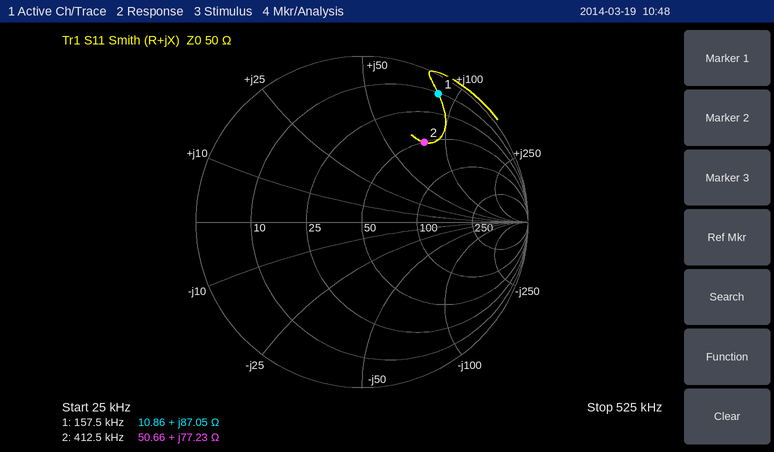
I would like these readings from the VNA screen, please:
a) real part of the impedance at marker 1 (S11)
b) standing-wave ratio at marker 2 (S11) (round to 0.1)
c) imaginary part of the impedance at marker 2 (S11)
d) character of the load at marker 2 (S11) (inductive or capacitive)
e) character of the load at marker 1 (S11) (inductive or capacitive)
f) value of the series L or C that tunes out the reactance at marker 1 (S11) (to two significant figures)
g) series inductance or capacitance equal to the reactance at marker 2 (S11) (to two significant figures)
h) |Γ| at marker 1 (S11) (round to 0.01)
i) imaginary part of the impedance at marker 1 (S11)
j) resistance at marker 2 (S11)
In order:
10.86 Ω
4.1
+77.23 Ω
inductive
inductive
12 nF
30 µH
0.90
+87.05 Ω
50.66 Ω
